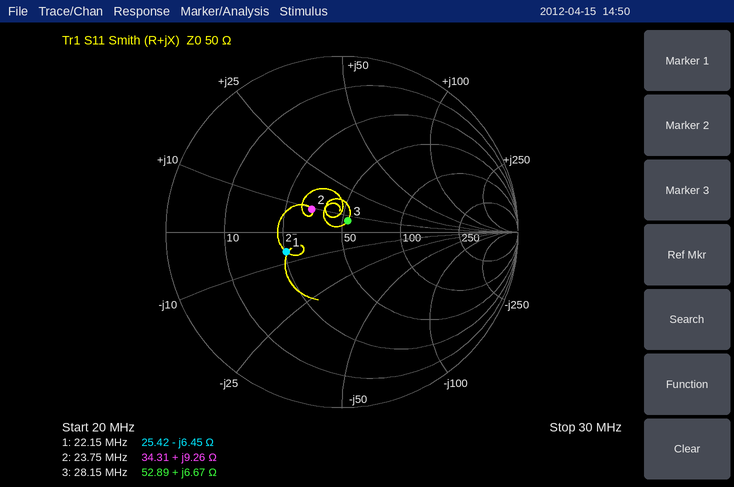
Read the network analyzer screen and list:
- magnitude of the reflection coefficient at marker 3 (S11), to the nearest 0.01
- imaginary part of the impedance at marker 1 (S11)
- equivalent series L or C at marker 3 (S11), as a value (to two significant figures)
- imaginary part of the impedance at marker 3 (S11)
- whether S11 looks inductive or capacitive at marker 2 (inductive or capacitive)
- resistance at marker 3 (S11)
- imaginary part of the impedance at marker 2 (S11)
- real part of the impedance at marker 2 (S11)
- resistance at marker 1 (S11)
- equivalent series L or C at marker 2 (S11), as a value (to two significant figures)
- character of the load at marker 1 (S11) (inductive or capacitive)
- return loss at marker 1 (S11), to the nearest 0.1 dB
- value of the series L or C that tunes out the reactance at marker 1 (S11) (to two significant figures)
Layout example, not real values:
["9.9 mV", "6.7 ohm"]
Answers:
["0.07", "-6.45 Ω", "38 nH", "+6.67 Ω", "inductive", "52.89 Ω", "+9.26 Ω", "34.31 Ω", "25.42 Ω", "62 nH", "capacitive", "9.5 dB", "46 nH"]
